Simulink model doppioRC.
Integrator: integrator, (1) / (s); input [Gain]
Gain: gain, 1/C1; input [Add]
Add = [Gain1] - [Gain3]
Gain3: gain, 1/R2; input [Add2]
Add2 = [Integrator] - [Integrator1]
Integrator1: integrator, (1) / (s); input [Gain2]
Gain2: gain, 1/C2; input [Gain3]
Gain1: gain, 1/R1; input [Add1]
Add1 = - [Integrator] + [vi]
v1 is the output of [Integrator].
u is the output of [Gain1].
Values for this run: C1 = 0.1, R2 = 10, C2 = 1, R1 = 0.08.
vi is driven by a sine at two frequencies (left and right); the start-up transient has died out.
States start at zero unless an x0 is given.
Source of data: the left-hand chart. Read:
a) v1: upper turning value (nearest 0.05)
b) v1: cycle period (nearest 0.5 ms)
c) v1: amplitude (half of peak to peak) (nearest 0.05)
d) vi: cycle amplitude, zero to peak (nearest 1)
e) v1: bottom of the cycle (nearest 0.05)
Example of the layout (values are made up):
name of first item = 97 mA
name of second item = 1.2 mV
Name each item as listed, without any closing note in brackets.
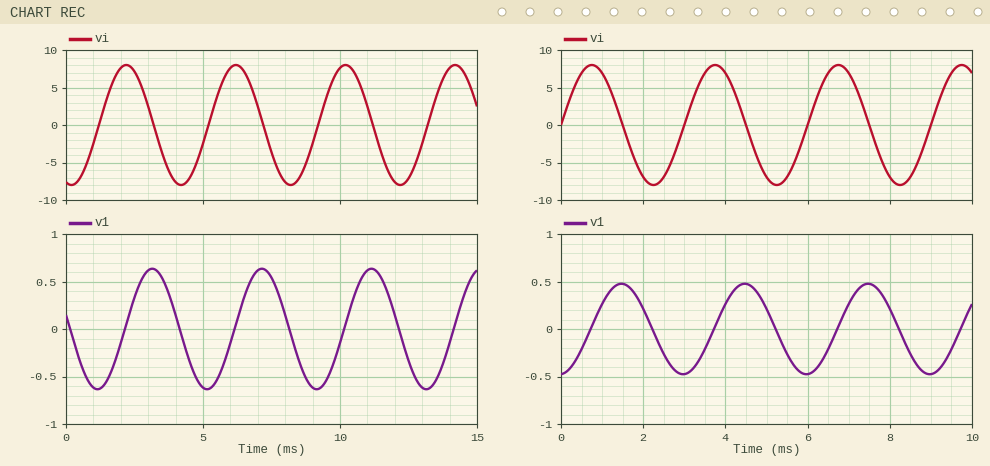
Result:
v1: upper turning value = 0.65
v1: cycle period = 4.0 ms
v1: amplitude (half of peak to peak) = 0.65
vi: cycle amplitude, zero to peak = 8
v1: bottom of the cycle = -0.65
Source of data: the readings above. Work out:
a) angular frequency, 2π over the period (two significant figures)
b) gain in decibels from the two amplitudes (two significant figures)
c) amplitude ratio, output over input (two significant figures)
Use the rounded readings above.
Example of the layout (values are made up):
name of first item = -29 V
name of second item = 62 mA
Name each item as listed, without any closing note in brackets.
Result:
angular frequency, 2π over the period = 1.6 rad/ms
gain in decibels from the two amplitudes = -22 dB
amplitude ratio, output over input = 0.081
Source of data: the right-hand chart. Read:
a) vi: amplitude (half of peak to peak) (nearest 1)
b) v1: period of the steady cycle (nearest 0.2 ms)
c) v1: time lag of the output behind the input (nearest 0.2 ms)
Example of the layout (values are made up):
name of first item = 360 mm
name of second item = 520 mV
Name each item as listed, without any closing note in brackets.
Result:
vi: amplitude (half of peak to peak) = 8
v1: period of the steady cycle = 3.0 ms
v1: time lag of the output behind the input = 0.8 ms
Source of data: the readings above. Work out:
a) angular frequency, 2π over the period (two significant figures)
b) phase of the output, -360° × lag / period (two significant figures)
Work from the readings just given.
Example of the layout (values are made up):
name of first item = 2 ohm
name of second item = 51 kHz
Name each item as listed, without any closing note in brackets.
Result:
angular frequency, 2π over the period = 2.1 rad/ms
phase of the output, -360° × lag / period = -96°
